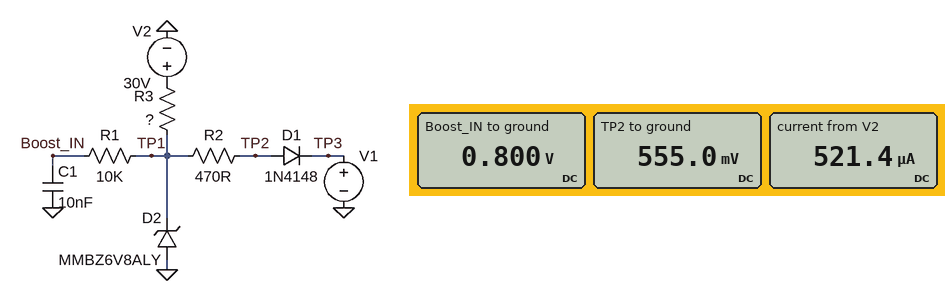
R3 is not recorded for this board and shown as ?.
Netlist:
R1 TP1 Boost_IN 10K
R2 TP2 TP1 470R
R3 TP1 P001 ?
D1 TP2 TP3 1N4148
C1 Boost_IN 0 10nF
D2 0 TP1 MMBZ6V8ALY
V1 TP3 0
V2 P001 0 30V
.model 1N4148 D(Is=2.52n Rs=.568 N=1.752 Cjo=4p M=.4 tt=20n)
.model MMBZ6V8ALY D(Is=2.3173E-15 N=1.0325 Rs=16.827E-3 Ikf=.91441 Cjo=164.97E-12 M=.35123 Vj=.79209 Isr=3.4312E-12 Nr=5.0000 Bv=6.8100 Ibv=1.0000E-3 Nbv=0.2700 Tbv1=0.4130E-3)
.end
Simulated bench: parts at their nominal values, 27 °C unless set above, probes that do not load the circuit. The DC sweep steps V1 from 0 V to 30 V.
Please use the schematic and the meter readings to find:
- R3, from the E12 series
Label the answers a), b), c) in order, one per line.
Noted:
a) 56 kΩ
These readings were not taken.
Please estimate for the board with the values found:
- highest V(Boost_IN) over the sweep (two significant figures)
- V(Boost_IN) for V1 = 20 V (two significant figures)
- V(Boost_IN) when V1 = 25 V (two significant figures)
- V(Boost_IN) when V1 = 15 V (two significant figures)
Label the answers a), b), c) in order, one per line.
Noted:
a) 6.8 V
b) 6.8 V
c) 6.8 V
d) 6.8 V
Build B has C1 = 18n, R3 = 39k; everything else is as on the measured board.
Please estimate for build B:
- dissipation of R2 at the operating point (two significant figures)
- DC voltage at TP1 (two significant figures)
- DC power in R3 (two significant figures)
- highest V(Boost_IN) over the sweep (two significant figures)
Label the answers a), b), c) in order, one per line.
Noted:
a) 260 µW
b) 920 mV
c) 22 mW
d) 6.8 V
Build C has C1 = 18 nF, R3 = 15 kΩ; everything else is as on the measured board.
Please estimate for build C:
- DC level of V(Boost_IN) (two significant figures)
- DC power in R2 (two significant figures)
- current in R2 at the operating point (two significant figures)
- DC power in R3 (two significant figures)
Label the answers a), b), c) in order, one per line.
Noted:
a) 1.5 V
b) 1.7 mW
c) 1.9 mA
d) 54 mW
